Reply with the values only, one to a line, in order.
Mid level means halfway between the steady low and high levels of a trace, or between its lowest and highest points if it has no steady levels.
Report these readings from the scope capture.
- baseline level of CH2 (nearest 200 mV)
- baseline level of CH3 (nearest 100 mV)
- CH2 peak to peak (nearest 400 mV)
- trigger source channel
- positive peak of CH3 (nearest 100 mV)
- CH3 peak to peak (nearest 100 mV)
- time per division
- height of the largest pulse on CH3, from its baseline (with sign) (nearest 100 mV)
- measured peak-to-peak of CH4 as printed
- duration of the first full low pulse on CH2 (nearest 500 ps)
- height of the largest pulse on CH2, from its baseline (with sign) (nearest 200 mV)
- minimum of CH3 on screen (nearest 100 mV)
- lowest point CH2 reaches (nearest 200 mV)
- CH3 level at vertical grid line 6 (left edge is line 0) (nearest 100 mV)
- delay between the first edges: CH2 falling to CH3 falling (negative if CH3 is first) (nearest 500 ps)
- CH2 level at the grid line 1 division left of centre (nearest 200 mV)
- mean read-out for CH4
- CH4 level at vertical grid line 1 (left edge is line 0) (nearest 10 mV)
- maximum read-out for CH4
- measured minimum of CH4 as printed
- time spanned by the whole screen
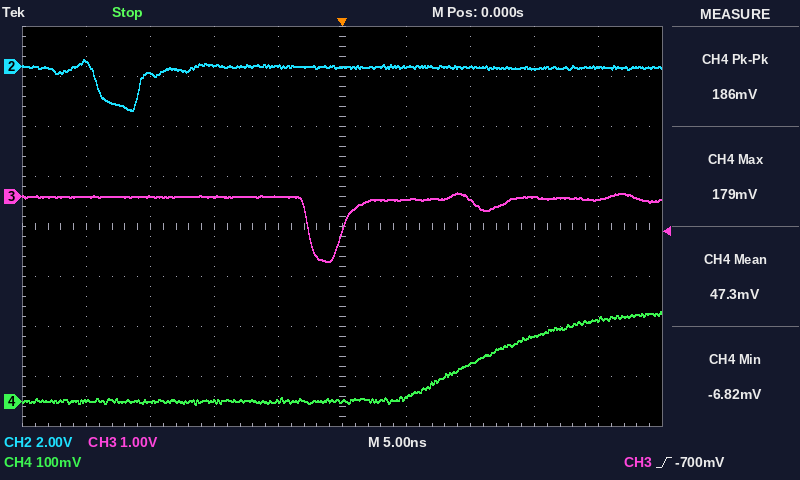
0.0 V
0.0 V
2.0 V
CH3
100 mV
1.4 V
5 ns
-1.3 V
186 mV
3.5 ns
-1.8 V
-1.3 V
-1.8 V
-100 mV
+16.5 ns
0.0 V
47.3 mV
0 mV
179 mV
-6.82 mV
50 ns
